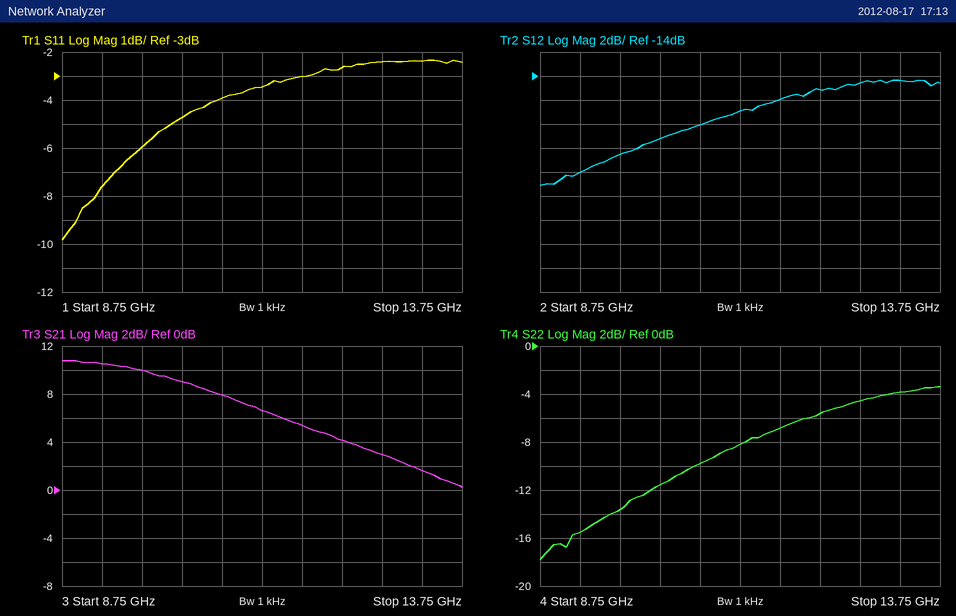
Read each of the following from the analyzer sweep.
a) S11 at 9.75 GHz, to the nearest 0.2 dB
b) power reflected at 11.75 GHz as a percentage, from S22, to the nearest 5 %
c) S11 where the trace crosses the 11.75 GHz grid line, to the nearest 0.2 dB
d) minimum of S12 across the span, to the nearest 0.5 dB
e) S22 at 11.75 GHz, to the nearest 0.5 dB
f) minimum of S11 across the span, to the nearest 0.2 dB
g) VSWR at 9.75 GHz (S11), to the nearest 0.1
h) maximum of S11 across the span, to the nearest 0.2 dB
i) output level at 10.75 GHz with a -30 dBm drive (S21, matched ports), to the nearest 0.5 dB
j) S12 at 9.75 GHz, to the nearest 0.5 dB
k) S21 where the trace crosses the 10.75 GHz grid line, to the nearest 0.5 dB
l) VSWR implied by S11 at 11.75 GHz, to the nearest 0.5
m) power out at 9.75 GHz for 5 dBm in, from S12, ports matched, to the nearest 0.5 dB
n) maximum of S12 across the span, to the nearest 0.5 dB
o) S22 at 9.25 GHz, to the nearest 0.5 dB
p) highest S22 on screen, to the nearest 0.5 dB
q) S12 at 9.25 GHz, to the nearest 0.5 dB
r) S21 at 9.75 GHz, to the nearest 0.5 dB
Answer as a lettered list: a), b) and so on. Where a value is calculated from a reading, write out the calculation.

a) -6.0 dB
b) 10^(-7/10) ≈ 20 %
c) -3.0 dB
d) -23.0 dB
e) -7.0 dB
f) -9.8 dB
g) |Γ| = 10^(-6/20) = 0.5012; VSWR = (1 + 0.5012)/(1 − 0.5012) ≈ 3.0
h) -2.4 dB
i) -30 dBm + (8.0 dB) = -22.0 dBm
j) -20.5 dB
k) 8.0 dB
l) |Γ| = 10^(-3/20) = 0.7079; VSWR = (1 + 0.7079)/(1 − 0.7079) ≈ 5.85, so 6.0 to the nearest 0.5
m) 5 dBm + (-20.5 dB) = -15.5 dBm
n) -14.5 dB
o) -15.5 dB
p) -3.5 dB
q) -22.0 dB
r) 10.0 dB
